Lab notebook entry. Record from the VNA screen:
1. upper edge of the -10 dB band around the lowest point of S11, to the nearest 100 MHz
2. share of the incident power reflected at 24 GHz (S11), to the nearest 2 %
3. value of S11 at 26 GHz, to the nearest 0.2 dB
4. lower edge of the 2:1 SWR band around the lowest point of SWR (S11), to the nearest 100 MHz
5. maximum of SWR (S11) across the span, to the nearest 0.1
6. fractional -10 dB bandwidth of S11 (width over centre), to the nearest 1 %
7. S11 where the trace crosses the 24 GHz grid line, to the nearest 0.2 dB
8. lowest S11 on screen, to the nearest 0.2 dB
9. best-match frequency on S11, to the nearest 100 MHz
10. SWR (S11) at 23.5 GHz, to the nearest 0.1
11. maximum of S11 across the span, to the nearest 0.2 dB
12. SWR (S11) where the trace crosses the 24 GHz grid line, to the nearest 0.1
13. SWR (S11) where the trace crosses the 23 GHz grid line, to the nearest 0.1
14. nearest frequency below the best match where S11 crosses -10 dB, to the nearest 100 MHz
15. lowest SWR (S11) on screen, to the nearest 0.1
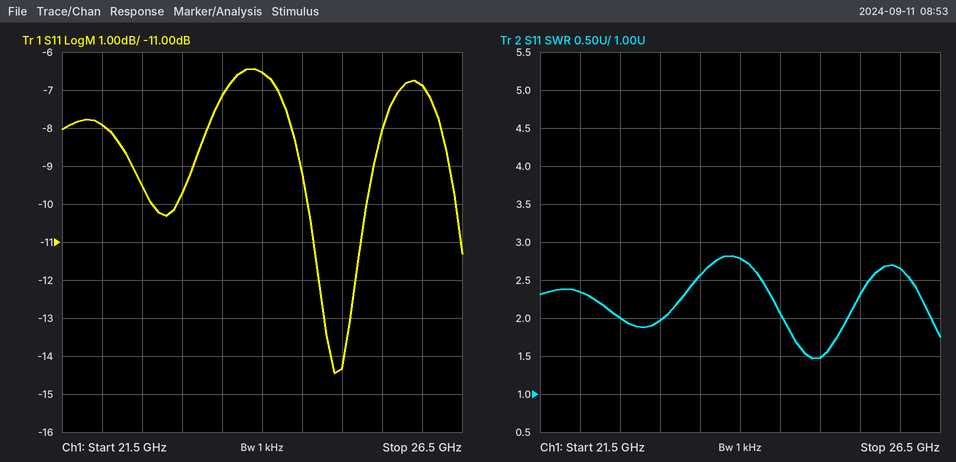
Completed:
25.3 GHz
22 %
-6.8 dB
24.5 GHz
2.8
3 %
-6.6 dB
-14.4 dB
24.9 GHz
2.6
-6.4 dB
2.8
2.0
24.6 GHz
1.5
